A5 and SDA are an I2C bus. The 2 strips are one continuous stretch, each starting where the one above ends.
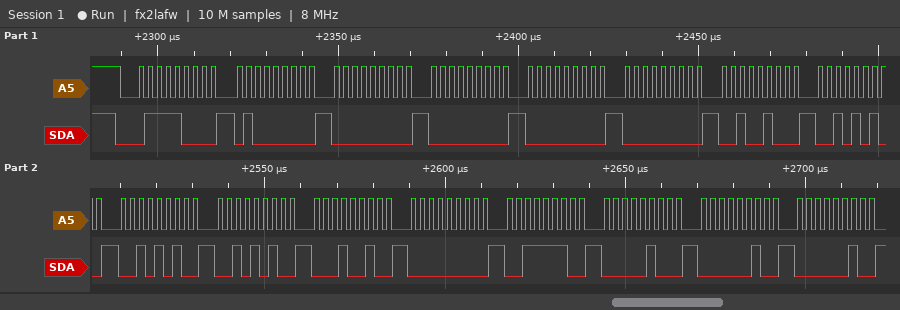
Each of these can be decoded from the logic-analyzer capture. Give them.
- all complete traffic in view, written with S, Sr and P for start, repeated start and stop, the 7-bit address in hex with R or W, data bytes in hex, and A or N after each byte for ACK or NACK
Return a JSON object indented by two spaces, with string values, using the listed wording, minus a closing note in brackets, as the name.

{
  "all complete traffic in view, written with S, Sr and P for start, repeated start and stop, the 7-bit address in hex with R or W, data bytes in hex, and A or N after each byte for ACK or NACK": "S 3CW A 40 A 00 A 00 A 00 A 00 A 24 A 2A A 2A A 2A A 12 A 00 A 3E A 04 A 02 A 02 A"
}
